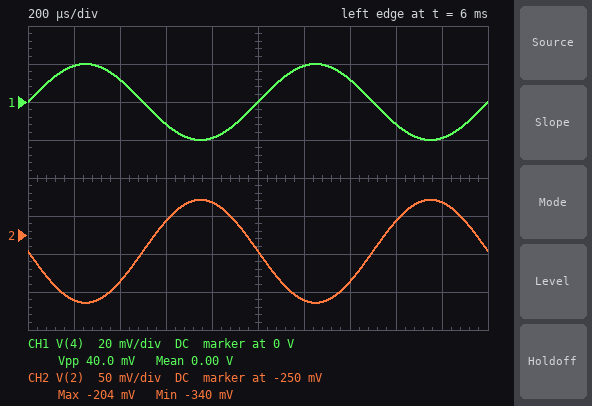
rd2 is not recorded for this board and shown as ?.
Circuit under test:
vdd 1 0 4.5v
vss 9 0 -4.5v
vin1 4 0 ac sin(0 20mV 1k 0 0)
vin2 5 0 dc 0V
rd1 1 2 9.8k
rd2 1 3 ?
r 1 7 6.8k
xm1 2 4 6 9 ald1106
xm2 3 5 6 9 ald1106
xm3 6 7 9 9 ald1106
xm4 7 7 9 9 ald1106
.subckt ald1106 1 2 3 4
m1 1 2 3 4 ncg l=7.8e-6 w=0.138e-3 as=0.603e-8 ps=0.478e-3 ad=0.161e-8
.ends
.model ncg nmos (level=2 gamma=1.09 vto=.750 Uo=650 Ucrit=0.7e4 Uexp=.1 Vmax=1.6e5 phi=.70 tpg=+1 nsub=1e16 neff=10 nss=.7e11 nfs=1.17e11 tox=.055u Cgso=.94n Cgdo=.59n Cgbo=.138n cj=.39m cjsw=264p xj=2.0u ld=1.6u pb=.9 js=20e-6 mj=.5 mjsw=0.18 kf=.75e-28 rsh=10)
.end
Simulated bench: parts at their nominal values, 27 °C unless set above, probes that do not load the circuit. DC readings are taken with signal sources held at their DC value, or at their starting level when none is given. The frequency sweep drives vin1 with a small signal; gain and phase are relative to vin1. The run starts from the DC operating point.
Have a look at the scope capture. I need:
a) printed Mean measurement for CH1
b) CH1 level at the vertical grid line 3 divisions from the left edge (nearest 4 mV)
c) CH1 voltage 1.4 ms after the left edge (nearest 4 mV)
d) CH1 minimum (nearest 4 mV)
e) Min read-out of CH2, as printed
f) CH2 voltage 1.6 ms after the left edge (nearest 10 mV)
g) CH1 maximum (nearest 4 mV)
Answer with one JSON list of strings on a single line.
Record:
["0.00 V", "-12 mV", "12 mV", "-20 mV", "-340 mV", "-230 mV", "20 mV"]
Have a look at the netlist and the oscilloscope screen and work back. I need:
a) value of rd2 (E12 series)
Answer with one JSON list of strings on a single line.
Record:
["12 kΩ"]
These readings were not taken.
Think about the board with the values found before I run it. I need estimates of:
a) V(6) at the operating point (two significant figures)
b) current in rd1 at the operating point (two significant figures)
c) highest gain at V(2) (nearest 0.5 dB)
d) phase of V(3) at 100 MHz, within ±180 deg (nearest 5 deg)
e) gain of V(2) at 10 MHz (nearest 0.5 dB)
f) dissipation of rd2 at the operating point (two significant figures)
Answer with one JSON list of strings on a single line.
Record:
["-2.5 V", "490 µA", "11.0 dB", "-100 deg", "10.5 dB", "2.7 mW"]
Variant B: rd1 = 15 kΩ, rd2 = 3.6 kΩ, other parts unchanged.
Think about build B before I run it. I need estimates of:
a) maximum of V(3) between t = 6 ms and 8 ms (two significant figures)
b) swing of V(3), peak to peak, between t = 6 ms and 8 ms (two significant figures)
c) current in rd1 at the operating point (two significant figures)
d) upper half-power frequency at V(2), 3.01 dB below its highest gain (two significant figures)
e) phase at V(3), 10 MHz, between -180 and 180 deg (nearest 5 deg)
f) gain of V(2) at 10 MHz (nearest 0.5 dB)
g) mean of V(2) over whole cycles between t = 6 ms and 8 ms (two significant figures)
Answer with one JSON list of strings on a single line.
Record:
["2.6 V", "12 mV", "430 µA", "69 MHz", "20 deg", "1.0 dB", "-1.9 V"]
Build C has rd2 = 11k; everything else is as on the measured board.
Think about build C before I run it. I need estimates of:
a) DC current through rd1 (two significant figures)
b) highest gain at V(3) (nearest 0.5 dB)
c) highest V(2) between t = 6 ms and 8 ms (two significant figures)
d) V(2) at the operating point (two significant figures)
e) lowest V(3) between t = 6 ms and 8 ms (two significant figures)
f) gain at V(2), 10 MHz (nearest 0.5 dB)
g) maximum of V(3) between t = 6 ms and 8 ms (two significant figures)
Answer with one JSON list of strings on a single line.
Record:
["480 µA", "11.5 dB", "-170 mV", "-240 mV", "-800 mV", "11.0 dB", "-650 mV"]
